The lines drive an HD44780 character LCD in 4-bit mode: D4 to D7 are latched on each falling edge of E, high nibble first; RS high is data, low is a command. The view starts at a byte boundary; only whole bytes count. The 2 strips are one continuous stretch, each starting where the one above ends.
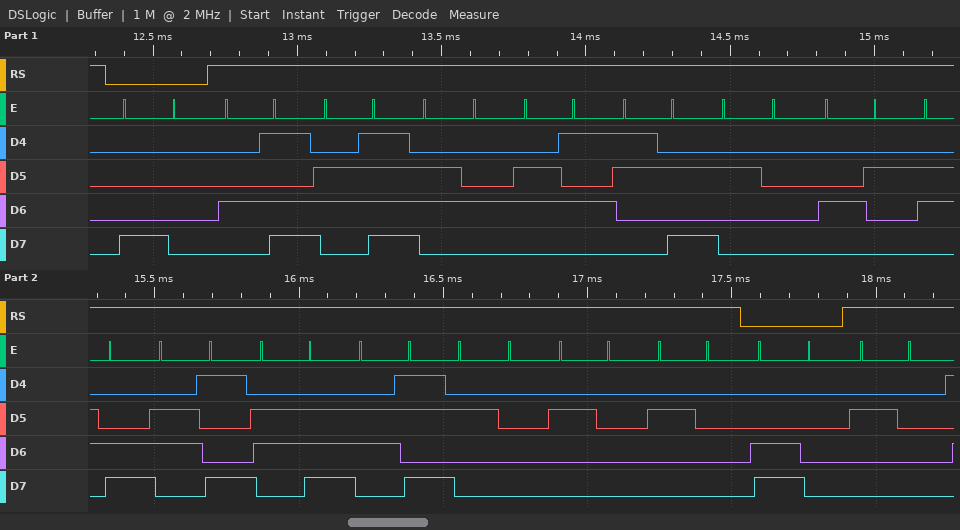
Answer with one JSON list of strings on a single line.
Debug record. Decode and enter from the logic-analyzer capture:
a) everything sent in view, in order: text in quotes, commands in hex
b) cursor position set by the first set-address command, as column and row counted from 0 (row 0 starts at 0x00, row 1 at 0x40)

["0x80 \"Mode: Blink   \" 0xC0 \" \"", "column 0, row 0"]
